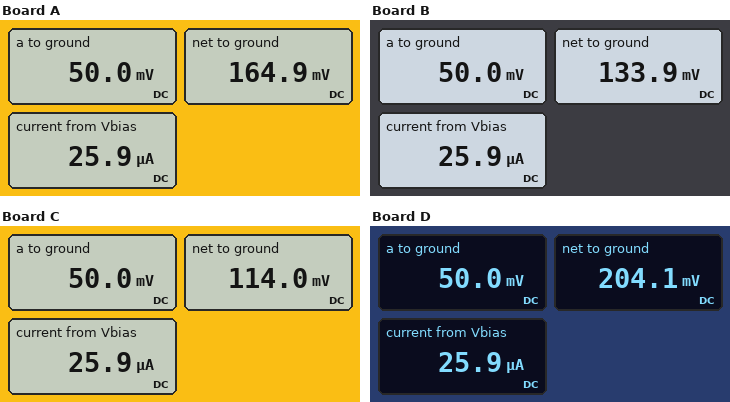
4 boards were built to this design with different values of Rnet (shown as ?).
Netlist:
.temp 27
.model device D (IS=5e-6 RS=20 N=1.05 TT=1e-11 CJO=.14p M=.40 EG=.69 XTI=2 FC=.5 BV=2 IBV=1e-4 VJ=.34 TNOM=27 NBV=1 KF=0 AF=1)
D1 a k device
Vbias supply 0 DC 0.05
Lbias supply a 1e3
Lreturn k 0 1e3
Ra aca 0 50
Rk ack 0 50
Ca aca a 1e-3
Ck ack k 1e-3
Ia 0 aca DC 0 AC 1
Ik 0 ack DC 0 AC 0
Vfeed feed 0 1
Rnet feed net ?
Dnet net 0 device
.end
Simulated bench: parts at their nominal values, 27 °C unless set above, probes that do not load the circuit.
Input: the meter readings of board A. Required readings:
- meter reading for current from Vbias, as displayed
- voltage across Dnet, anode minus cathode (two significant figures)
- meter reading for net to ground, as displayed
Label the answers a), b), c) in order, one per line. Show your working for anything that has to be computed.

a) 25.9 µA
b) 164.9 mV = 160 mV
c) 164.9 mV
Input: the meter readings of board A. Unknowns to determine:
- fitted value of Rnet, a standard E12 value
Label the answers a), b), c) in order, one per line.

a) 820 Ω
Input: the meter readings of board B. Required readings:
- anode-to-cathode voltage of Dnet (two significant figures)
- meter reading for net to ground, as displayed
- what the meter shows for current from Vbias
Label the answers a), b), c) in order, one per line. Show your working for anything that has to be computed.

a) 133.9 mV = 130 mV
b) 133.9 mV
c) 25.9 µA
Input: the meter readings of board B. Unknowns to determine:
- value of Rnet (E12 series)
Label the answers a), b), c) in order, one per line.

a) 1.8 kΩ
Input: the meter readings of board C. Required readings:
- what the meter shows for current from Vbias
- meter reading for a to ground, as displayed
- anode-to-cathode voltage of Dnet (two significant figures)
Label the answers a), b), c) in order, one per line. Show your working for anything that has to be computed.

a) 25.9 µA
b) 50.0 mV
c) 114 mV = 110 mV
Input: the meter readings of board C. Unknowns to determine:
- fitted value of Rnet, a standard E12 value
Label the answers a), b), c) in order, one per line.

a) 3.3 kΩ
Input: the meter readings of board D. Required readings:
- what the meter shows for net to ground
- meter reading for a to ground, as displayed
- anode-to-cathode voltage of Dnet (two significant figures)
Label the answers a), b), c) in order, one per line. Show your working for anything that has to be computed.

a) 204.1 mV
b) 50.0 mV
c) 204.1 mV = 200 mV
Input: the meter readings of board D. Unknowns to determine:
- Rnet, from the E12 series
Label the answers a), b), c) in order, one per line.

a) 390 Ω
